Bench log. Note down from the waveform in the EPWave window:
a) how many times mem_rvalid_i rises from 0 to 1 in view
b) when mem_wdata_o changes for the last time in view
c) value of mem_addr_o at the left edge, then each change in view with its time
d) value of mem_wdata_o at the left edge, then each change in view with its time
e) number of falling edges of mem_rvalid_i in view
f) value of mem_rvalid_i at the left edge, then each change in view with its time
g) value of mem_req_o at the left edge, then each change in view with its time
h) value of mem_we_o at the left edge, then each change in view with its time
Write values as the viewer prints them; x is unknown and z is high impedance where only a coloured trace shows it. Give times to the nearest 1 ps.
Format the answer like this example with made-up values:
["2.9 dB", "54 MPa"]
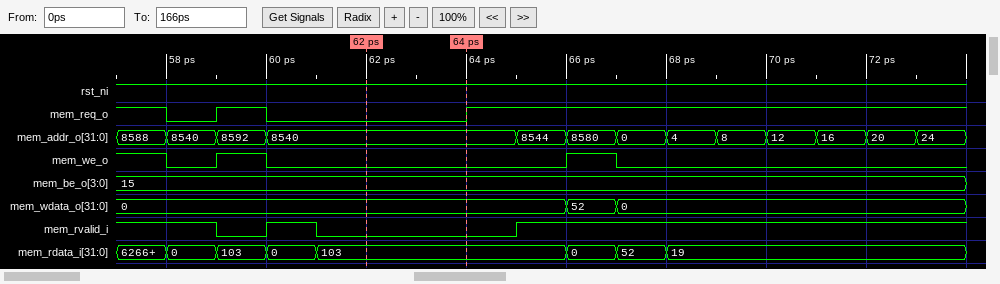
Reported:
["2", "67 ps", "8588, 8540 at 58 ps, 8592 at 59 ps, 8540 at 60 ps, 8544 at 65 ps, 8580 at 66 ps, 0 at 67 ps, 4 at 68 ps, 8 at 69 ps, 12 at 70 ps, 16 at 71 ps, 20 at 72 ps, 24 at 73 ps", "0, 52 at 66 ps, 0 at 67 ps", "2", "1, 0 at 59 ps, 1 at 60 ps, 0 at 61 ps, 1 at 65 ps", "1, 0 at 58 ps, 1 at 59 ps, 0 at 60 ps, 1 at 64 ps", "1, 0 at 58 ps, 1 at 59 ps, 0 at 60 ps, 1 at 66 ps, 0 at 67 ps"]
